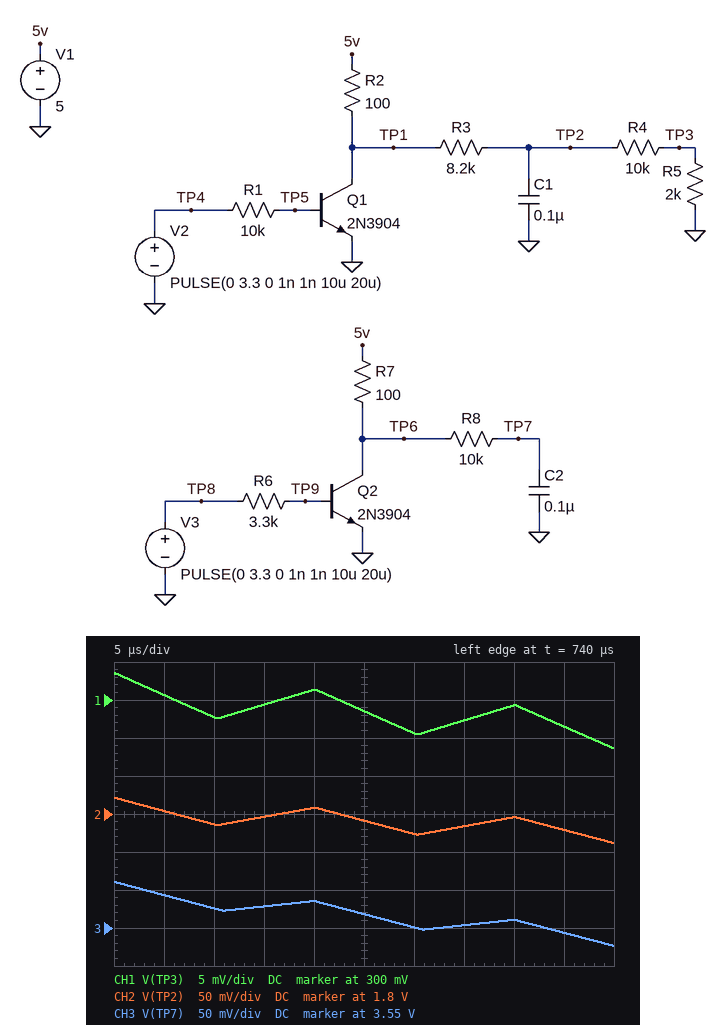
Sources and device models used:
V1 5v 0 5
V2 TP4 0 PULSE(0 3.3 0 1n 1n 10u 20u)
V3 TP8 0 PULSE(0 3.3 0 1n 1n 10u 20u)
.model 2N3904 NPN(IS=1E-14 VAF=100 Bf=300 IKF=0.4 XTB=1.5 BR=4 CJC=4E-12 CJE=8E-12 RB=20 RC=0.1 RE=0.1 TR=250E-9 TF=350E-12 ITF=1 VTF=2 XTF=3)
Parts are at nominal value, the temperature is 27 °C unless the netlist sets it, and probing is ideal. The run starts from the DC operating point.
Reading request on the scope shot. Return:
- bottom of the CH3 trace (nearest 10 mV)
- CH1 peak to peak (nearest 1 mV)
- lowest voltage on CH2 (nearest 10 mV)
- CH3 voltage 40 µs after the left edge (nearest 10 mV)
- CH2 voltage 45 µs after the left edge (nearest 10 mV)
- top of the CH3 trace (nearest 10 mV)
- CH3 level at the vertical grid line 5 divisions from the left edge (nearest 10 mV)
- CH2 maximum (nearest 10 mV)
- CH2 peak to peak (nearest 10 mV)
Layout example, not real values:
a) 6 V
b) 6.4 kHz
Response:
a) 3.53 V
b) 10 mV
c) 1.76 V
d) 3.56 V
e) 1.78 V
f) 3.61 V
g) 3.57 V
h) 1.82 V
i) 60 mV
